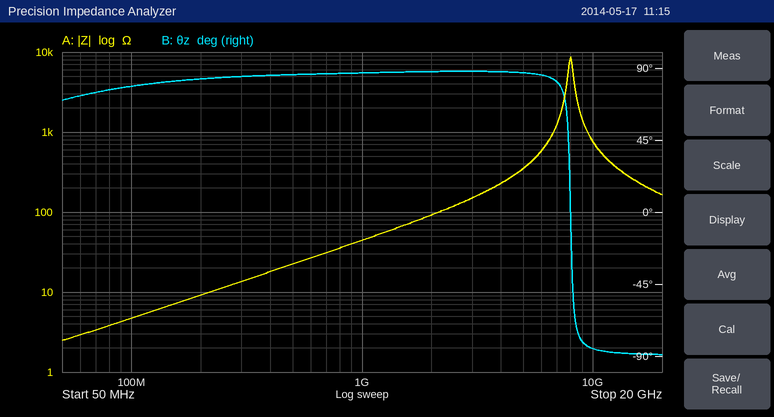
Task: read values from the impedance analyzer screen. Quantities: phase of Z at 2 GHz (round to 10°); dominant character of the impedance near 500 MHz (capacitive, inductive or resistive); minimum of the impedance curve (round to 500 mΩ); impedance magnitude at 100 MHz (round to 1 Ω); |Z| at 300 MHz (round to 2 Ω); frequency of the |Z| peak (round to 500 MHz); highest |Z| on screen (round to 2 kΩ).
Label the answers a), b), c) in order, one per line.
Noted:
a) 90°
b) inductive
c) 2.5 Ω
d) 5 Ω
e) 14 Ω
f) 8.0 GHz
g) 8 kΩ
